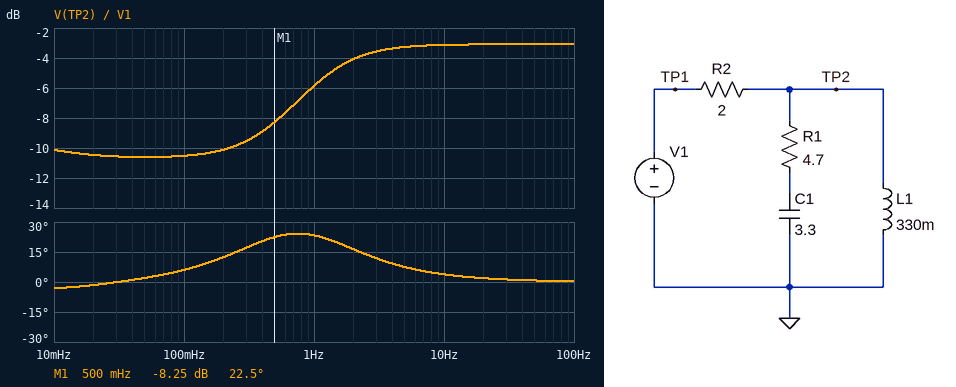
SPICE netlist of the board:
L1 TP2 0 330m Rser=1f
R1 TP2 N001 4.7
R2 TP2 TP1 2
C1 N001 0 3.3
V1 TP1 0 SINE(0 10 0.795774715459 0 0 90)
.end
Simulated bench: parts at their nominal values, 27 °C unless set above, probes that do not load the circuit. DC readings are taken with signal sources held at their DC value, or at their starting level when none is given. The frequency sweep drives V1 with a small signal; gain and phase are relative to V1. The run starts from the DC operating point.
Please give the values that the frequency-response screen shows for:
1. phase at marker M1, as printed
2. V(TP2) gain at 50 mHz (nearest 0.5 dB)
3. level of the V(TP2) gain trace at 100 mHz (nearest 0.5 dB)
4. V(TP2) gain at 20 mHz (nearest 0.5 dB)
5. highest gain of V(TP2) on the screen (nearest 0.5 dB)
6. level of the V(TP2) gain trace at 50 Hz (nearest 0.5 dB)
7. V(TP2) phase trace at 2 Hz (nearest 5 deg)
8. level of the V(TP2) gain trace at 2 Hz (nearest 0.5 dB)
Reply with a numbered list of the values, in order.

1. 22.5 deg
2. -10.5 dB
3. -10.5 dB
4. -10.5 dB
5. -3.0 dB
6. -3.0 dB
7. 15 deg
8. -4.0 dB
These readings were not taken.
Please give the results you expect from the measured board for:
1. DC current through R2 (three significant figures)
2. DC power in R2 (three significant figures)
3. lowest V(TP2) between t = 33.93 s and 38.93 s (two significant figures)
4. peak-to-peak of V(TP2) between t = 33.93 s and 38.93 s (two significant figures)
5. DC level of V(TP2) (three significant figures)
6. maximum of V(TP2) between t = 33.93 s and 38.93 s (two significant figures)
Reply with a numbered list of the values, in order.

1. 3.33 A
2. 22.2 W
3. -4.6 V
4. 9.3 V
5. 3.33 V
6. 4.7 V
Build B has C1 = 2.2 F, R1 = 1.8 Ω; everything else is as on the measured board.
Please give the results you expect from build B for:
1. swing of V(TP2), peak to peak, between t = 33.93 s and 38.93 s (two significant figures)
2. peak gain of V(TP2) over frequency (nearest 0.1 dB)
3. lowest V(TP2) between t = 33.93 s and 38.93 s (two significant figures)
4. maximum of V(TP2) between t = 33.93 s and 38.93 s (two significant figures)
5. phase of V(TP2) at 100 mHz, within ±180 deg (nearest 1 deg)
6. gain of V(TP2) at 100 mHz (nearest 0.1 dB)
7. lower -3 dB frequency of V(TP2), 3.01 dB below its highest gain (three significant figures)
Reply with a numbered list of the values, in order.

1. 7.2 V
2. -6.5 dB
3. -3.6 V
4. 3.6 V
5. 0 deg
6. -11.8 dB
7. 628 mHz
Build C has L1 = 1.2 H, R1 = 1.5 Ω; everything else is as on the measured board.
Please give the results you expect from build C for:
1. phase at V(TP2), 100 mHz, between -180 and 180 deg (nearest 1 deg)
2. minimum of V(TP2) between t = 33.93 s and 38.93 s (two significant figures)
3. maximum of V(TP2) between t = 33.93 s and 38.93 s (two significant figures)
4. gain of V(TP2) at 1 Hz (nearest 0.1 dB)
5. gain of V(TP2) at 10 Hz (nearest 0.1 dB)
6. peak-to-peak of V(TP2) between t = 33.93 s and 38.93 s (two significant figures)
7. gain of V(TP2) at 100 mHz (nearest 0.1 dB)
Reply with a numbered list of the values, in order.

1. 9 deg
2. -4.2 V
3. 4.2 V
4. -7.5 dB
5. -7.4 dB
6. 8.3 V
7. -11.0 dB
